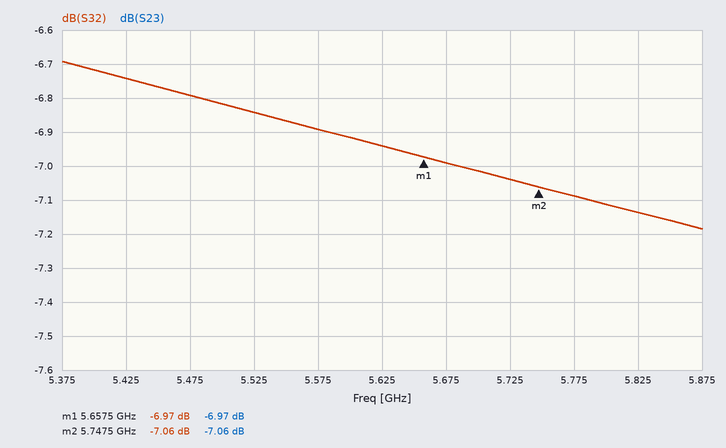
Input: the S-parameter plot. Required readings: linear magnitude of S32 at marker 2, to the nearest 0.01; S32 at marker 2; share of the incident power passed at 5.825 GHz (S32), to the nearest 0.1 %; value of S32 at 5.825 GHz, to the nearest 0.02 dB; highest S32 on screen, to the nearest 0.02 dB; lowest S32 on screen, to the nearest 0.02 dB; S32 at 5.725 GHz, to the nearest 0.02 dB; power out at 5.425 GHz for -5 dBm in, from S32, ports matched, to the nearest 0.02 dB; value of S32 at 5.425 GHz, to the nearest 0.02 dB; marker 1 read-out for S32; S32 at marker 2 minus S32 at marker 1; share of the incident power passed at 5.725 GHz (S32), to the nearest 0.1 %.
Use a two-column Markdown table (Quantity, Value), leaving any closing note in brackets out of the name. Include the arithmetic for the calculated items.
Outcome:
| Quantity | Value |
|---|---|
| linear magnitude of S32 at marker 2, to the nearest 0.01 | 10^(-7.06/20) ≈ 0.44 |
| S32 at marker 2 | -7.06 dB |
| share of the incident power passed at 5.825 GHz (S32), to the nearest 0.1 % | 10^(-7.14/10) ≈ 19.3 % |
| value of S32 at 5.825 GHz, to the nearest 0.02 dB | -7.14 dB |
| highest S32 on screen, to the nearest 0.02 dB | -6.70 dB |
| lowest S32 on screen, to the nearest 0.02 dB | -7.18 dB |
| S32 at 5.725 GHz, to the nearest 0.02 dB | -7.04 dB |
| power out at 5.425 GHz for -5 dBm in, from S32, ports matched, to the nearest 0.02 dB | -5 dBm + (-6.74 dB) = -11.74 dBm |
| value of S32 at 5.425 GHz, to the nearest 0.02 dB | -6.74 dB |
| marker 1 read-out for S32 | -6.97 dB |
| S32 at marker 2 minus S32 at marker 1 | -7.06 − (-6.97) = -0.09 dB |
| share of the incident power passed at 5.725 GHz (S32), to the nearest 0.1 % | 10^(-7.04/10) ≈ 19.8 % |
